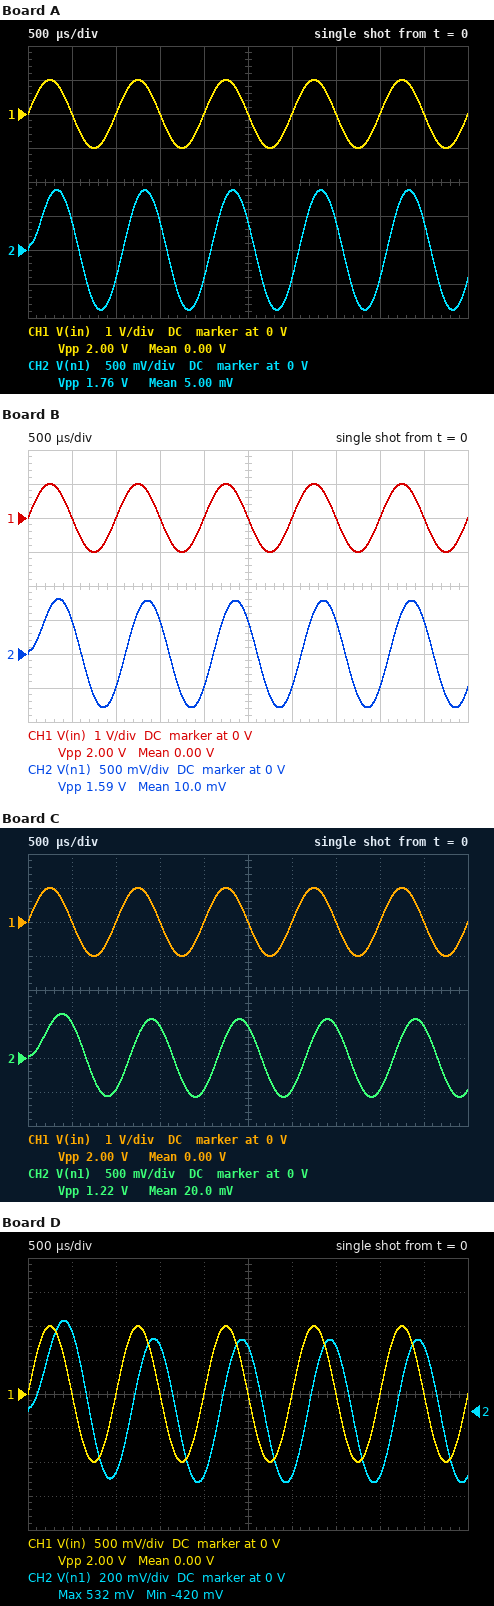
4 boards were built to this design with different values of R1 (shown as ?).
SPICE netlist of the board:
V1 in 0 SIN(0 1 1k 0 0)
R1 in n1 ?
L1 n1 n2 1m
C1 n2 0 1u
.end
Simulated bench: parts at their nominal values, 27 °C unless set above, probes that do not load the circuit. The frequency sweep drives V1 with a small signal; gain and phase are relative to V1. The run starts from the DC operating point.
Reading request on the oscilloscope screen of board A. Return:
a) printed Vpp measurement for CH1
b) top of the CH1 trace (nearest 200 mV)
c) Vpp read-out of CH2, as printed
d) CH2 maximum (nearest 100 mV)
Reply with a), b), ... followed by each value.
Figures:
a) 2.00 V
b) 1.0 V
c) 1.76 V
d) 900 mV
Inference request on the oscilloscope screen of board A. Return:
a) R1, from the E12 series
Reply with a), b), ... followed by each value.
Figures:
a) 82 Ω
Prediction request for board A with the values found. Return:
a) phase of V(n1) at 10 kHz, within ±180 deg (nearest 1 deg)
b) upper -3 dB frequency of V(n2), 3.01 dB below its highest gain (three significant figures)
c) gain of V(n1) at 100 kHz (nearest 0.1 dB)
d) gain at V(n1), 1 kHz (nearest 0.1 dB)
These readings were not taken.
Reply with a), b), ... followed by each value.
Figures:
a) 60 deg
b) 2.27 kHz
c) -0.1 dB
d) -1.1 dB
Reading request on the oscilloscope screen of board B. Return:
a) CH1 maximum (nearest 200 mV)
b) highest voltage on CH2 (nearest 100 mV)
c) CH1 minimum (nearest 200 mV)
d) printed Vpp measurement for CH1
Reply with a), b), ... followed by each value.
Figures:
a) 1.0 V
b) 800 mV
c) -1.0 V
d) 2.00 V
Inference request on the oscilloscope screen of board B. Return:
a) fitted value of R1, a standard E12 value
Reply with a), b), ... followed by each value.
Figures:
a) 120 Ω
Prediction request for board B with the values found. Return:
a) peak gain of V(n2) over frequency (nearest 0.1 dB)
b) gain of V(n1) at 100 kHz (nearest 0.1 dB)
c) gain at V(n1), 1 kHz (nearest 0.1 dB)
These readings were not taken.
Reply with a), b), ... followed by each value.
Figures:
a) 0 dB
b) -0.2 dB
c) -2.1 dB
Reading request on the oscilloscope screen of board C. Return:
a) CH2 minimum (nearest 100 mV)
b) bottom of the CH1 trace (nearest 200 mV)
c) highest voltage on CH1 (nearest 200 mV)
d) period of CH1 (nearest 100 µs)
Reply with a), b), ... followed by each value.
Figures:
a) -600 mV
b) -1.0 V
c) 1.0 V
d) 1.0 ms
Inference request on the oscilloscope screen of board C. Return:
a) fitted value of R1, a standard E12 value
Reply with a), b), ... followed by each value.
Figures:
a) 220 Ω
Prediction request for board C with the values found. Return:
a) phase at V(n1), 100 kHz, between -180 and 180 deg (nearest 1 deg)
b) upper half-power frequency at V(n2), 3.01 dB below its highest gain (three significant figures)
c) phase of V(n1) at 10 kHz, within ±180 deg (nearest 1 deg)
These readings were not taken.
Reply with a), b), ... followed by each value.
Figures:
a) 19 deg
b) 739 Hz
c) 78 deg
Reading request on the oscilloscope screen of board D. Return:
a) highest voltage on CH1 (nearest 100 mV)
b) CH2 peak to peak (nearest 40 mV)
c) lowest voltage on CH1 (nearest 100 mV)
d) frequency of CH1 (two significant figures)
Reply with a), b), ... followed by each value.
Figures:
a) 1.0 V
b) 960 mV
c) -1.0 V
d) 1.0 kHz
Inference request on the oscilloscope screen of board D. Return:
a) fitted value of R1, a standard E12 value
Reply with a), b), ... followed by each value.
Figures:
a) 330 Ω
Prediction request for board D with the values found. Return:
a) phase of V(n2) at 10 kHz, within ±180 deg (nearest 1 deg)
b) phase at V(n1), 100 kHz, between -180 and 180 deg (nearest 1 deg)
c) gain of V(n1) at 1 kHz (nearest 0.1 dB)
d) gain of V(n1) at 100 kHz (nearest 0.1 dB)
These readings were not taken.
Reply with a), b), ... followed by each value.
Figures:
a) -98 deg
b) 28 deg
c) -7.5 dB
d) -1.1 dB
